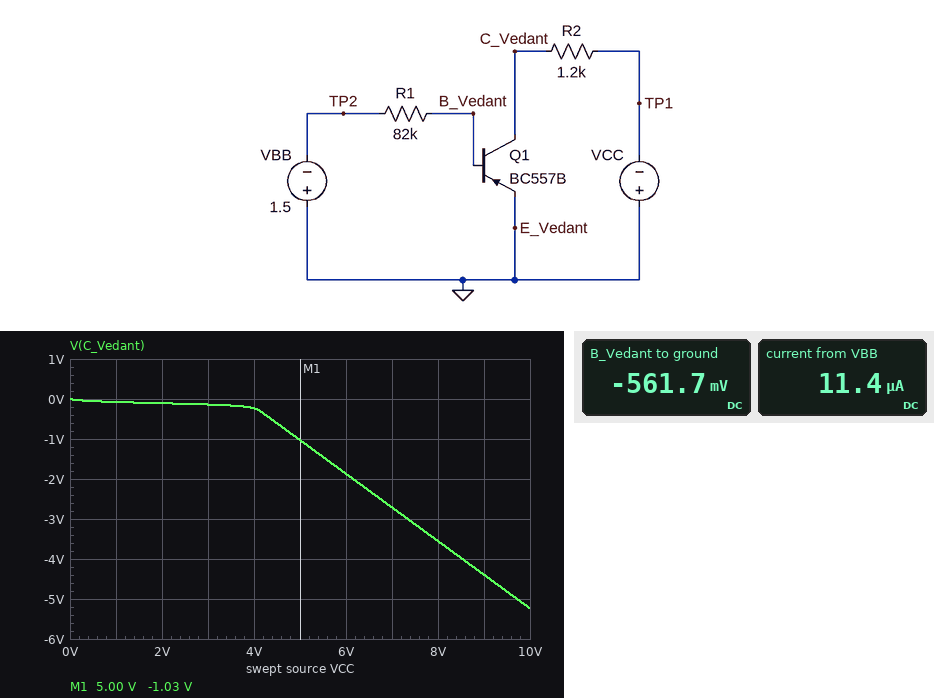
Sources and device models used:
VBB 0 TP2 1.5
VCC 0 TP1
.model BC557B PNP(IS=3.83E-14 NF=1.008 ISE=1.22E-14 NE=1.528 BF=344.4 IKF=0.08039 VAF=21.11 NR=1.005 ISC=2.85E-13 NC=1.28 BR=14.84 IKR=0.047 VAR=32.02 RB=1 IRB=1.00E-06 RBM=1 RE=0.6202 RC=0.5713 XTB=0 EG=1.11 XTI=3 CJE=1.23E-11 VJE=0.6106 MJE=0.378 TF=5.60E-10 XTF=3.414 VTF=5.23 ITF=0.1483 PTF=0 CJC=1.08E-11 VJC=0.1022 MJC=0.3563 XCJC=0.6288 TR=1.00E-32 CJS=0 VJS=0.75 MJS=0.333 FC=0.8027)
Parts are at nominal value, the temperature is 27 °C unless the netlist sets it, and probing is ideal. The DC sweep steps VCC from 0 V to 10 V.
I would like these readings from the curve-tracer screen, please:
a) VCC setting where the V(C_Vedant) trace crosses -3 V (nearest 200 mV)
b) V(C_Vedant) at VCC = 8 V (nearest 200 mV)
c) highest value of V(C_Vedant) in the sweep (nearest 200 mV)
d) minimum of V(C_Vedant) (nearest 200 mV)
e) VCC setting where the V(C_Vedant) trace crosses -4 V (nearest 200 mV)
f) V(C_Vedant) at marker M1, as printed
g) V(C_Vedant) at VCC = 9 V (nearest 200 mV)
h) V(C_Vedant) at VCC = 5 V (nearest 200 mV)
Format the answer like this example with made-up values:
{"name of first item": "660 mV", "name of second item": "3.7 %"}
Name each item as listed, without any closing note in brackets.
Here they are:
{"VCC setting where the V(C_Vedant) trace crosses -3 V": "7.4 V", "V(C_Vedant) at VCC = 8 V": "-3.6 V", "highest value of V(C_Vedant) in the sweep": "0 V", "minimum of V(C_Vedant)": "-5.2 V", "VCC setting where the V(C_Vedant) trace crosses -4 V": "8.6 V", "V(C_Vedant) at marker M1, as printed": "-1.03 V", "V(C_Vedant) at VCC = 9 V": "-4.4 V", "V(C_Vedant) at VCC = 5 V": "-1.0 V"}
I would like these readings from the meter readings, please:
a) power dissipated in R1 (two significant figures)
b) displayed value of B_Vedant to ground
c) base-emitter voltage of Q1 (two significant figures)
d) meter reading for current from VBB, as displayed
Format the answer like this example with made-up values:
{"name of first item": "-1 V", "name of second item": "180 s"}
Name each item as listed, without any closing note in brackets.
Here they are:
{"power dissipated in R1": "11 µW", "displayed value of B_Vedant to ground": "-561.7 mV", "base-emitter voltage of Q1": "-560 mV", "meter reading for current from VBB, as displayed": "11.4 µA"}
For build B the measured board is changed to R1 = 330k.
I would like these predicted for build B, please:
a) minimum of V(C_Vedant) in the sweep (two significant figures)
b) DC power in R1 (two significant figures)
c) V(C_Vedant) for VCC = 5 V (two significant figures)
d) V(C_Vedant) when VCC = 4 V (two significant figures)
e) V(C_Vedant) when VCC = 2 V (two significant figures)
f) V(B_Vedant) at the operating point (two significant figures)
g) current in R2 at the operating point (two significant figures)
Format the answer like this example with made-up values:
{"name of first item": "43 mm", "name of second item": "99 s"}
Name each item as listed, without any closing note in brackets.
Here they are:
{"minimum of V(C_Vedant) in the sweep": "-8.6 V", "DC power in R1": "2.9 µW", "V(C_Vedant) for VCC = 5 V": "-3.8 V", "V(C_Vedant) when VCC = 4 V": "-2.9 V", "V(C_Vedant) when VCC = 2 V": "-950 mV", "V(B_Vedant) at the operating point": "-520 mV", "current in R2 at the operating point": "2.2 µA"}
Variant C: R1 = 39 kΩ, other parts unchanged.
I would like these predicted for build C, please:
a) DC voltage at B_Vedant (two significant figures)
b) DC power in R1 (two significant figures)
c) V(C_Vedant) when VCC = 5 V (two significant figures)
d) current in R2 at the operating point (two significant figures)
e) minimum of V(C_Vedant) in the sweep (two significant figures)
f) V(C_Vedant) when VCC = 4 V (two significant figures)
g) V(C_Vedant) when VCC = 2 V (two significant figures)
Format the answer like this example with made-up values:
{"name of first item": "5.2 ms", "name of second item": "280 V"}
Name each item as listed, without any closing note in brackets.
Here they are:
{"DC voltage at B_Vedant": "-580 mV", "DC power in R1": "22 µW", "V(C_Vedant) when VCC = 5 V": "-120 mV", "current in R2 at the operating point": "3.8 µA", "minimum of V(C_Vedant) in the sweep": "-1.8 V", "V(C_Vedant) when VCC = 4 V": "-110 mV", "V(C_Vedant) when VCC = 2 V": "-75 mV"}
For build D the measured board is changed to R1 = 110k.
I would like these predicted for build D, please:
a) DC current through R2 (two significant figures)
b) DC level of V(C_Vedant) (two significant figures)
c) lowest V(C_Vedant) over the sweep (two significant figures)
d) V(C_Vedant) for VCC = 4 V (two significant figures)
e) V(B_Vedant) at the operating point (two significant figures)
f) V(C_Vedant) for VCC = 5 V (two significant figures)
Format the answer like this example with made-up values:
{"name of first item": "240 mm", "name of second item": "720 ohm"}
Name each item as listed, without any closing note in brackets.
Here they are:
{"DC current through R2": "3.3 µA", "DC level of V(C_Vedant)": "-4.0 mV", "lowest V(C_Vedant) over the sweep": "-6.2 V", "V(C_Vedant) for VCC = 4 V": "-990 mV", "V(B_Vedant) at the operating point": "-550 mV", "V(C_Vedant) for VCC = 5 V": "-1.9 V"}
